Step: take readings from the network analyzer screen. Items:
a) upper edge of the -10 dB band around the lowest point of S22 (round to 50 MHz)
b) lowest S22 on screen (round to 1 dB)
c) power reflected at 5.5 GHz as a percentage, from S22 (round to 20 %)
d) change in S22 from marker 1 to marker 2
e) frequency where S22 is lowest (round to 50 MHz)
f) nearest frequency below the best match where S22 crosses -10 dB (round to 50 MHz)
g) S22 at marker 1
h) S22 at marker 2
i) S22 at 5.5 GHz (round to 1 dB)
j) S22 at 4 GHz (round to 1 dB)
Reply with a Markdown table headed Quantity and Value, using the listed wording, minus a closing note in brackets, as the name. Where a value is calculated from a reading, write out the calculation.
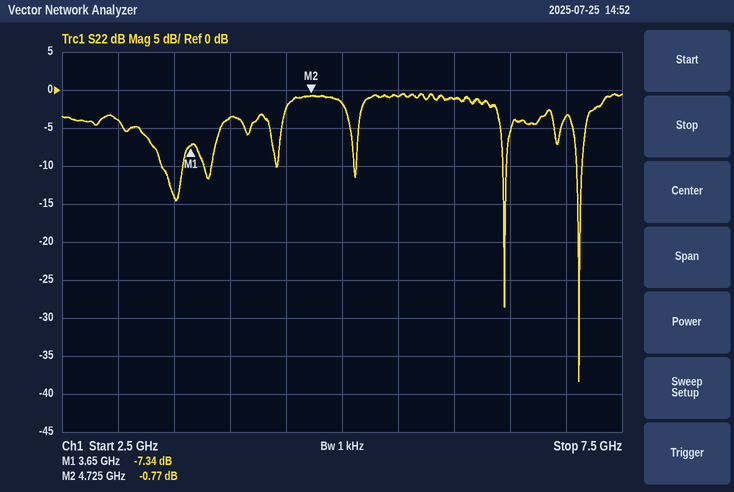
| Quantity | Value |
|---|---|
| upper edge of the -10 dB band around the lowest point of S22 | 7.15 GHz |
| lowest S22 on screen | -38 dB |
| power reflected at 5.5 GHz as a percentage, from S22 | 10^(-1/10) ≈ 79.4 %, so 80 % to the nearest 20 % |
| change in S22 from marker 1 to marker 2 | -0.77 − (-7.34) = 6.57 dB |
| frequency where S22 is lowest | 7.10 GHz |
| nearest frequency below the best match where S22 crosses -10 dB | 7.10 GHz |
| S22 at marker 1 | -7.34 dB |
| S22 at marker 2 | -0.77 dB |
| S22 at 5.5 GHz | -1 dB |
| S22 at 4 GHz | -4 dB |
